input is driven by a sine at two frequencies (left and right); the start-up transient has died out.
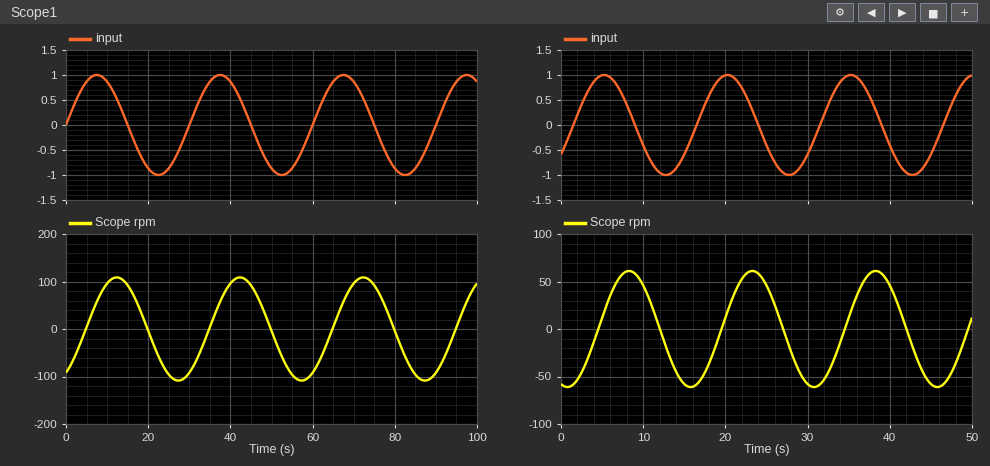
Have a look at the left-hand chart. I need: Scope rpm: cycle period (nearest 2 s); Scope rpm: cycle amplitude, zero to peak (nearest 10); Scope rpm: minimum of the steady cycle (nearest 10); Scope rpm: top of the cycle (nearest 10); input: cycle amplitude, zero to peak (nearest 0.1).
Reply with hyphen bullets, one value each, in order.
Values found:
- 30 s
- 110
- -110
- 110
- 1.0
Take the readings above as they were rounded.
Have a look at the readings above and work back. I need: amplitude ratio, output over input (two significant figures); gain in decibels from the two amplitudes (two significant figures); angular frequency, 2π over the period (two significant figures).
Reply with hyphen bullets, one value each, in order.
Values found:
- 110
- 41 dB
- 0.21 rad/s
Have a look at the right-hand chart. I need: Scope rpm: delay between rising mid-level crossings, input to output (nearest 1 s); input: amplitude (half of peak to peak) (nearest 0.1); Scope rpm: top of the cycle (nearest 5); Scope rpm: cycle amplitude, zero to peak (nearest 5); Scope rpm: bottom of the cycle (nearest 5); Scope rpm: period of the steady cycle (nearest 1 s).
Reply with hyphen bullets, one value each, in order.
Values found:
- 3 s
- 1.0
- 60
- 60
- -60
- 15 s
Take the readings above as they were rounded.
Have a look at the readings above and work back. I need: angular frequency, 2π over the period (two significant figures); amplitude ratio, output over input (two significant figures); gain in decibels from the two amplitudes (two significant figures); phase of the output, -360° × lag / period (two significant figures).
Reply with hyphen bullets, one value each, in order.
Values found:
- 0.42 rad/s
- 60
- 36 dB
- -72°
